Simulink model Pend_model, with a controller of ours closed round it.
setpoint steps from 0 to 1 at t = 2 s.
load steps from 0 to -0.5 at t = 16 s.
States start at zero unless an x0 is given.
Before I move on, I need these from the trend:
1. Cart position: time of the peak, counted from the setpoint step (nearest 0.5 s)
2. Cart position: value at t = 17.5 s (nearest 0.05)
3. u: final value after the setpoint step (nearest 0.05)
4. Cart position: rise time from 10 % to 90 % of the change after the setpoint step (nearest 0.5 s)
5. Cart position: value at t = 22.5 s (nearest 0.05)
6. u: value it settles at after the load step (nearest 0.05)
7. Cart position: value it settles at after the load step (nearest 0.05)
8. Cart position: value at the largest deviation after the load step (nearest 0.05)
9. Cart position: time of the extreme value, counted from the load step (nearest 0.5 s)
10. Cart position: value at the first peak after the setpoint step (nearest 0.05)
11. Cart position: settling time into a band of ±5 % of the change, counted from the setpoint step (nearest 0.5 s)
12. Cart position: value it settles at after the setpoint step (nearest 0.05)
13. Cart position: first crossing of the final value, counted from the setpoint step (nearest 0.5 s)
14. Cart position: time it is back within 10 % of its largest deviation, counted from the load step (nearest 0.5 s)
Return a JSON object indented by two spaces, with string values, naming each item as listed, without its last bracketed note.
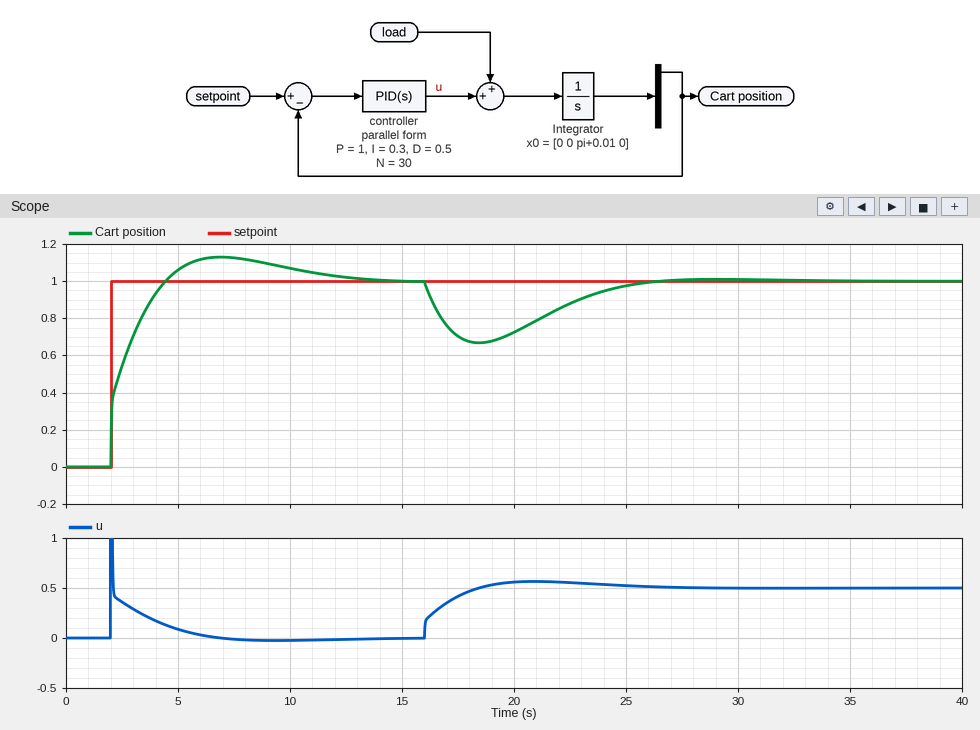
{
  "Cart position: time of the peak, counted from the setpoint step": "5.0 s",
  "Cart position: value at t = 17.5 s": "0.70",
  "u: final value after the setpoint step": "0.00",
  "Cart position: rise time from 10 % to 90 % of the change after the setpoint step": "2.0 s",
  "Cart position: value at t = 22.5 s": "0.90",
  "u: value it settles at after the load step": "0.50",
  "Cart position: value it settles at after the load step": "1.00",
  "Cart position: value at the largest deviation after the load step": "0.65",
  "Cart position: time of the extreme value, counted from the load step": "2.5 s",
  "Cart position: value at the first peak after the setpoint step": "1.15",
  "Cart position: settling time into a band of ±5 % of the change, counted from the setpoint step": "9.0 s",
  "Cart position: value it settles at after the setpoint step": "1.00",
  "Cart position: first crossing of the final value, counted from the setpoint step": "2.5 s",
  "Cart position: time it is back within 10 % of its largest deviation, counted from the load step": "8.5 s"
}
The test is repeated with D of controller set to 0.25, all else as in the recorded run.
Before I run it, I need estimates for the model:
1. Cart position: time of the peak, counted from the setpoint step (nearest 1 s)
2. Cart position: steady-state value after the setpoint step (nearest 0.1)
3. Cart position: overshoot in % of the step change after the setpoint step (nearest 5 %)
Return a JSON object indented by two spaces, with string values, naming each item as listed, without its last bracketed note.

{
  "Cart position: time of the peak, counted from the setpoint step": "4 s",
  "Cart position: steady-state value after the setpoint step": "1.0",
  "Cart position: overshoot in % of the step change after the setpoint step": "15 %"
}
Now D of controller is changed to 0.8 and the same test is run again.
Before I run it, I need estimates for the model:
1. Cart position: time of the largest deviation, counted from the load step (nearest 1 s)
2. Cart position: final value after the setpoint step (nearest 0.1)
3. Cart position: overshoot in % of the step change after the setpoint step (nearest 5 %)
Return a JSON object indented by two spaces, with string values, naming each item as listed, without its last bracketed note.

{
  "Cart position: time of the largest deviation, counted from the load step": "3 s",
  "Cart position: final value after the setpoint step": "1.0",
  "Cart position: overshoot in % of the step change after the setpoint step": "10 %"
}
